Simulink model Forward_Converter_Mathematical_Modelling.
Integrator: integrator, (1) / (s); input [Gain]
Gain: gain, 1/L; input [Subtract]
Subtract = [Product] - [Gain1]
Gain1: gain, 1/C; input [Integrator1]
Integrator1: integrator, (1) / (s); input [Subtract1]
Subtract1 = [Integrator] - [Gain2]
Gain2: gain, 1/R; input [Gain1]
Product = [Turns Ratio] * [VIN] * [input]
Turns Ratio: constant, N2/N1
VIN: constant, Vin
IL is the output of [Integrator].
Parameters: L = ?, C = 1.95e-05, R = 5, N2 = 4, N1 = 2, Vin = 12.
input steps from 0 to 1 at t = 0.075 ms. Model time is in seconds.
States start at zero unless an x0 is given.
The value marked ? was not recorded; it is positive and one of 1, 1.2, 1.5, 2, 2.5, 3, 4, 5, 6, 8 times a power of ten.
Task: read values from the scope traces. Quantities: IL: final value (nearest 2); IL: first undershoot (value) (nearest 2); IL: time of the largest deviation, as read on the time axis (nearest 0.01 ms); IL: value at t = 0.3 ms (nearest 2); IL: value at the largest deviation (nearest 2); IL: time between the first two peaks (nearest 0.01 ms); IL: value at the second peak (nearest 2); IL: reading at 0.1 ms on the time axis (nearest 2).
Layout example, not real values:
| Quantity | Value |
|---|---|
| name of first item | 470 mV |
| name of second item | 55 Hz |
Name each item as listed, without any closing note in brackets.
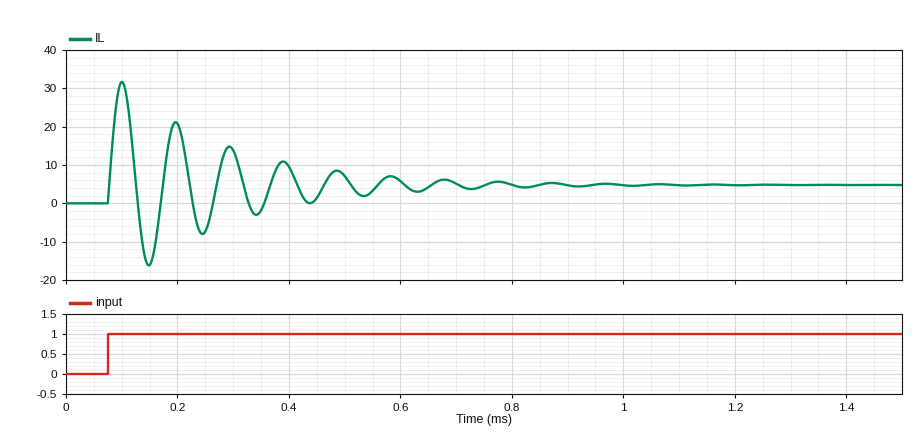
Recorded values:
| Quantity | Value |
|---|---|
| IL: final value | 4 |
| IL: first undershoot (value) | -16 |
| IL: time of the largest deviation, as read on the time axis | 0.10 ms |
| IL: value at t = 0.3 ms | 14 |
| IL: value at the largest deviation | 32 |
| IL: time between the first two peaks | 0.10 ms |
| IL: value at the second peak | 22 |
| IL: reading at 0.1 ms on the time axis | 32 |
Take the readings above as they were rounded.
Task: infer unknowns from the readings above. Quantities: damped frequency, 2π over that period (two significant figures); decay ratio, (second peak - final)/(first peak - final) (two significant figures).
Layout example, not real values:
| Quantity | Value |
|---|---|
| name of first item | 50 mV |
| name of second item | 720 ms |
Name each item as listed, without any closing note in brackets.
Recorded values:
| Quantity | Value |
|---|---|
| damped frequency, 2π over that period | 63 rad/ms |
| decay ratio, (second peak - final)/(first peak - final) | 0.64 |
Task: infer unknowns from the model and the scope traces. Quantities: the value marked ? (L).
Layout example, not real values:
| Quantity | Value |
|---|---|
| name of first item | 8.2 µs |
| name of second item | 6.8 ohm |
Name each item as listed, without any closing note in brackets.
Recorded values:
| Quantity | Value |
|---|---|
| the value marked ? | 1.2e-05 |
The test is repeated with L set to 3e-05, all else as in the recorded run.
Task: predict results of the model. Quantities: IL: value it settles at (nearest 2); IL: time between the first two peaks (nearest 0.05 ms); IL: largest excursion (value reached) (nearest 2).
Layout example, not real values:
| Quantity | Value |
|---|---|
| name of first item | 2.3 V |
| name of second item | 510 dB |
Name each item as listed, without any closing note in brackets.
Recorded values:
| Quantity | Value |
|---|---|
| IL: value it settles at | 4 |
| IL: time between the first two peaks | 0.15 ms |
| IL: largest excursion (value reached) | 20 |
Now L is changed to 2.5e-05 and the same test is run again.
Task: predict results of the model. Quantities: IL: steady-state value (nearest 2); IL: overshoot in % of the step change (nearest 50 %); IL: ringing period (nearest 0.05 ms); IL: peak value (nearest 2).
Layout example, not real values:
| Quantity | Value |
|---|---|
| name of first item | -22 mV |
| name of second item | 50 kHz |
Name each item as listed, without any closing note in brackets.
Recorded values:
| Quantity | Value |
|---|---|
| IL: steady-state value | 4 |
| IL: overshoot in % of the step change | 350 % |
| IL: ringing period | 0.15 ms |
| IL: peak value | 22 |
